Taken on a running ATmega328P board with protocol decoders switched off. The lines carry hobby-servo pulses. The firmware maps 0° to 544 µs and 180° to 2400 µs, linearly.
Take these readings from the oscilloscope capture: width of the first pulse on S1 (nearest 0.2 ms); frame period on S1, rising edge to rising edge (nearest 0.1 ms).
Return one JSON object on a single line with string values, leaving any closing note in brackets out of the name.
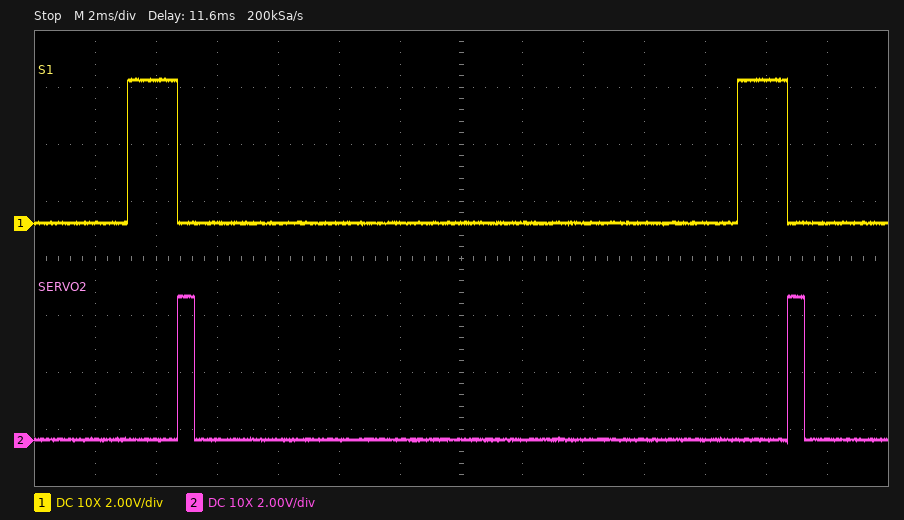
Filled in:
{"width of the first pulse on S1": "1.6 ms", "frame period on S1, rising edge to rising edge": "20.0 ms"}
